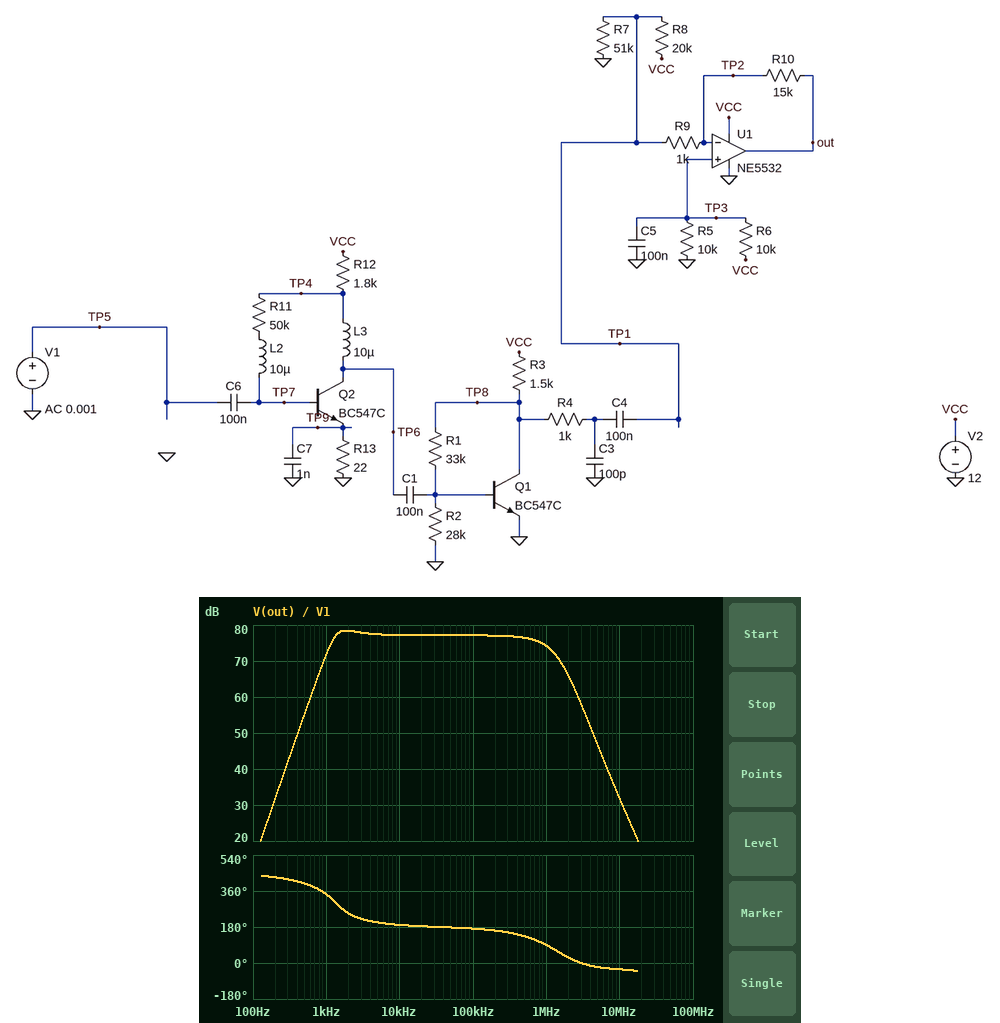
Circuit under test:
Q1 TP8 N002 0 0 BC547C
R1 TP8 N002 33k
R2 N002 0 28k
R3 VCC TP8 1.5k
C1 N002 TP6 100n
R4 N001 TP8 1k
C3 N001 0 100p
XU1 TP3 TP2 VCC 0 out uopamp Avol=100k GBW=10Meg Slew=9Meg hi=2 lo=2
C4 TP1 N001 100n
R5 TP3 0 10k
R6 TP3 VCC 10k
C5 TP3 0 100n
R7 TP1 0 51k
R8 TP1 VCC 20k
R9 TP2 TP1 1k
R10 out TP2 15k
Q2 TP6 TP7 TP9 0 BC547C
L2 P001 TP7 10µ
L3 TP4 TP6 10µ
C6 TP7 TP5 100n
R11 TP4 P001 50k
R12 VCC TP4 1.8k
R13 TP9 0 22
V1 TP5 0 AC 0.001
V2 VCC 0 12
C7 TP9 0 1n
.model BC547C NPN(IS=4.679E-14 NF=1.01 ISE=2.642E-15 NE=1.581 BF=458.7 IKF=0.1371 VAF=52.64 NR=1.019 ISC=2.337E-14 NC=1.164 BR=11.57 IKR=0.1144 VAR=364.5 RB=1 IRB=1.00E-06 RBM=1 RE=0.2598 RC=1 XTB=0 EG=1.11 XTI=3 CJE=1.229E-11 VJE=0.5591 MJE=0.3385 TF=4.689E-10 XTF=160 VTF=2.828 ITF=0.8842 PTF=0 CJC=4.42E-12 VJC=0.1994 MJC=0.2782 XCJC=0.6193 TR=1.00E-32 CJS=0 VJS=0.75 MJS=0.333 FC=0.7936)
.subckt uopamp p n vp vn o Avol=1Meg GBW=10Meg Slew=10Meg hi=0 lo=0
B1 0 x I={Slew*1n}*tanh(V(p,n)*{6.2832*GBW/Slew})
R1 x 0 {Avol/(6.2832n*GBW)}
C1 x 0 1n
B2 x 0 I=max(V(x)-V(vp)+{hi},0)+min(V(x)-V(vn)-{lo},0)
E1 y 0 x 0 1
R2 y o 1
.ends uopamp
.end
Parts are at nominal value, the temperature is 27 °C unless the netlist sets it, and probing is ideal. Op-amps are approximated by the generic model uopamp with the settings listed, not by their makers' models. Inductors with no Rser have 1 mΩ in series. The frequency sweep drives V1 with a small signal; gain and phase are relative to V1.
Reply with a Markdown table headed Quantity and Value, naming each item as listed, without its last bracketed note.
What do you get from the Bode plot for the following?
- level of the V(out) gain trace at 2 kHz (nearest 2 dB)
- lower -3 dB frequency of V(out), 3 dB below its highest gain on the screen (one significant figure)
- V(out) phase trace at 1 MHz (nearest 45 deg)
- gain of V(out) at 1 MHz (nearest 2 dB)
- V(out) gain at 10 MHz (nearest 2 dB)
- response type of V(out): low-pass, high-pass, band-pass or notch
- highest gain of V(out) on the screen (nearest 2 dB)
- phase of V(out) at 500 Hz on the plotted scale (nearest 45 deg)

| Quantity | Value |
|---|---|
| level of the V(out) gain trace at 2 kHz | 78 dB |
| lower -3 dB frequency of V(out), 3 dB below its highest gain on the screen | 1 kHz |
| V(out) phase trace at 1 MHz | 90 deg |
| gain of V(out) at 1 MHz | 74 dB |
| V(out) gain at 10 MHz | 32 dB |
| response type of V(out): low-pass, high-pass, band-pass or notch | band-pass |
| highest gain of V(out) on the screen | 78 dB |
| phase of V(out) at 500 Hz on the plotted scale | 405 deg |
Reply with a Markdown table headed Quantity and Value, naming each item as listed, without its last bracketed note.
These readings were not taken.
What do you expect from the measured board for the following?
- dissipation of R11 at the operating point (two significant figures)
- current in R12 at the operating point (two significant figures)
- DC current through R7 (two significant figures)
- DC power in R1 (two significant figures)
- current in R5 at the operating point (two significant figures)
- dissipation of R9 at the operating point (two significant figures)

| Quantity | Value |
|---|---|
| dissipation of R11 at the operating point | 8.7 µW |
| current in R12 at the operating point | 5.9 mA |
| DC current through R7 | 120 µA |
| DC power in R1 | 50 µW |
| current in R5 at the operating point | 600 µA |
| dissipation of R9 at the operating point | 29 µW |
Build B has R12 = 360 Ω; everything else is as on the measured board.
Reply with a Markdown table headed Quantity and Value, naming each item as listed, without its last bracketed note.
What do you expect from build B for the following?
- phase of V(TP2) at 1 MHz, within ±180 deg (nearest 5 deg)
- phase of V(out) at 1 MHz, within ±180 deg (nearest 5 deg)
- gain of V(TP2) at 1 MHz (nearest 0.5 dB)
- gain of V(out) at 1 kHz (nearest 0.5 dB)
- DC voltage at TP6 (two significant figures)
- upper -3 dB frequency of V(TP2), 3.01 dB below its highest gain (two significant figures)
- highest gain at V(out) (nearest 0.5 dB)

| Quantity | Value |
|---|---|
| phase of V(TP2) at 1 MHz, within ±180 deg | 10 deg |
| phase of V(out) at 1 MHz, within ±180 deg | 100 deg |
| gain of V(TP2) at 1 MHz | 53.5 dB |
| gain of V(out) at 1 kHz | 62.5 dB |
| DC voltage at TP6 | 3.9 V |
| upper -3 dB frequency of V(TP2), 3.01 dB below its highest gain | 2.3 MHz |
| highest gain at V(out) | 75.5 dB |
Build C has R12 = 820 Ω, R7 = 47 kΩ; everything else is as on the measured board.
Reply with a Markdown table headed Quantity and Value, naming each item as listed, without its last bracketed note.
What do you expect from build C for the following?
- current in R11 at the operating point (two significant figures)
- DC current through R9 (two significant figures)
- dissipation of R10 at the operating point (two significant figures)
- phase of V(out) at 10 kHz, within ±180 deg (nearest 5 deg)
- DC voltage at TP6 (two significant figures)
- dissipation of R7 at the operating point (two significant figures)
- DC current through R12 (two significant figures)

| Quantity | Value |
|---|---|
| current in R11 at the operating point | 27 µA |
| DC current through R9 | 160 µA |
| dissipation of R10 at the operating point | 390 µW |
| phase of V(out) at 10 kHz, within ±180 deg | -165 deg |
| DC voltage at TP6 | 2.3 V |
| dissipation of R7 at the operating point | 810 µW |
| DC current through R12 | 12 mA |
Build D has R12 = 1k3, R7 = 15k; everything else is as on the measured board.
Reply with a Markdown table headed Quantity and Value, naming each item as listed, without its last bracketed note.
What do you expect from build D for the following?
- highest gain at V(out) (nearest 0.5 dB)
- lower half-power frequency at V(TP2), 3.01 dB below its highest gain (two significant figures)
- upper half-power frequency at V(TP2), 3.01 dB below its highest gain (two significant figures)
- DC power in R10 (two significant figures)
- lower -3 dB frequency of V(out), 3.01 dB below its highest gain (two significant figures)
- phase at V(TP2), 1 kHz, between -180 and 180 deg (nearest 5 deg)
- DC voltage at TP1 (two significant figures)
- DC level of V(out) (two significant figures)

| Quantity | Value |
|---|---|
| highest gain at V(out) | 77.5 dB |
| lower half-power frequency at V(TP2), 3.01 dB below its highest gain | 570 kHz |
| upper half-power frequency at V(TP2), 3.01 dB below its highest gain | 2.2 MHz |
| DC power in R10 | 120 µW |
| lower -3 dB frequency of V(out), 3.01 dB below its highest gain | 1.3 kHz |
| phase at V(TP2), 1 kHz, between -180 and 180 deg | -115 deg |
| DC voltage at TP1 | 5.9 V |
| DC level of V(out) | 7.3 V |
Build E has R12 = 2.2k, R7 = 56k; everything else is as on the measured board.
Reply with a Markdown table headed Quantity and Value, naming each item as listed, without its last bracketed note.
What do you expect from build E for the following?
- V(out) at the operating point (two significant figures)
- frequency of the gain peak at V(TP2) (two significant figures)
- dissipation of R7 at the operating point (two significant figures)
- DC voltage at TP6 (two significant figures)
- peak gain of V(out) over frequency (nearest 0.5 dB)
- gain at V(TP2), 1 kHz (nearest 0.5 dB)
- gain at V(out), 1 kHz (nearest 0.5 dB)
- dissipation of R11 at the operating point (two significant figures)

| Quantity | Value |
|---|---|
| V(out) at the operating point | 3.3 V |
| frequency of the gain peak at V(TP2) | 1.2 MHz |
| dissipation of R7 at the operating point | 680 µW |
| DC voltage at TP6 | 1.3 V |
| peak gain of V(out) over frequency | 79.0 dB |
| gain at V(TP2), 1 kHz | -7.5 dB |
| gain at V(out), 1 kHz | 72.5 dB |
| dissipation of R11 at the operating point | 5.9 µW |
